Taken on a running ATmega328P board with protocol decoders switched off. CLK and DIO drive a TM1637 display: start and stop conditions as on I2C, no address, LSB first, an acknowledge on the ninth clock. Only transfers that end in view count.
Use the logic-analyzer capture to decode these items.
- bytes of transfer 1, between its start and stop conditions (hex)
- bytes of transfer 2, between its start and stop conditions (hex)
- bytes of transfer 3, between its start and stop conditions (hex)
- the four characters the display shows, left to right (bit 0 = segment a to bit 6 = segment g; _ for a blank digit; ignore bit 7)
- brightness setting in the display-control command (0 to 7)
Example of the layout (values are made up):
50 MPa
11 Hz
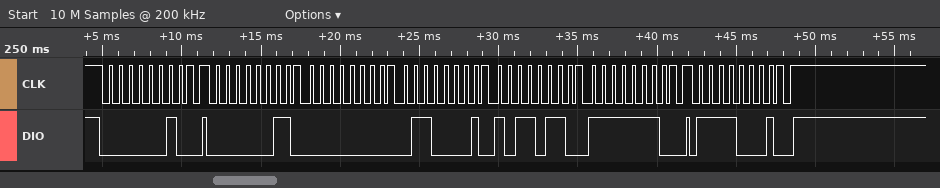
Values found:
40
C0 00 86 6D 7F
8F
_158
7
